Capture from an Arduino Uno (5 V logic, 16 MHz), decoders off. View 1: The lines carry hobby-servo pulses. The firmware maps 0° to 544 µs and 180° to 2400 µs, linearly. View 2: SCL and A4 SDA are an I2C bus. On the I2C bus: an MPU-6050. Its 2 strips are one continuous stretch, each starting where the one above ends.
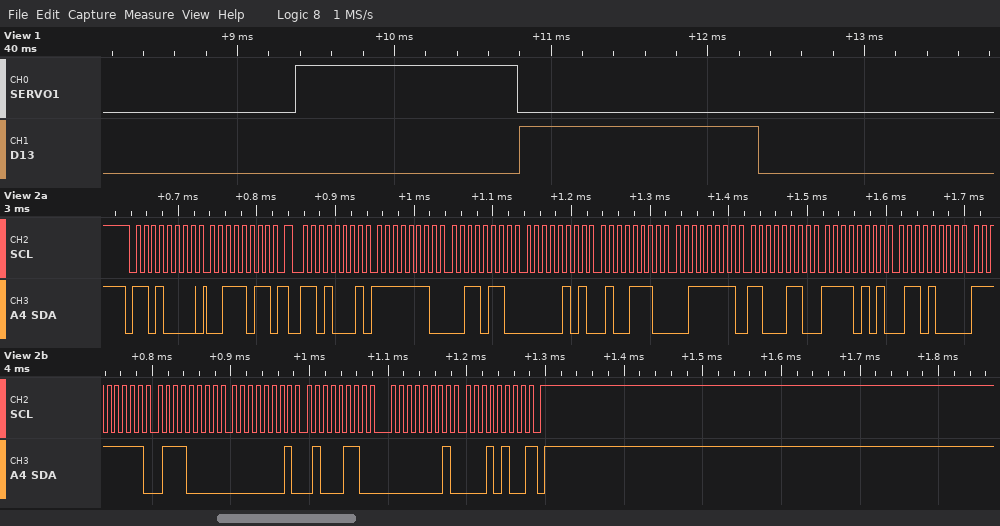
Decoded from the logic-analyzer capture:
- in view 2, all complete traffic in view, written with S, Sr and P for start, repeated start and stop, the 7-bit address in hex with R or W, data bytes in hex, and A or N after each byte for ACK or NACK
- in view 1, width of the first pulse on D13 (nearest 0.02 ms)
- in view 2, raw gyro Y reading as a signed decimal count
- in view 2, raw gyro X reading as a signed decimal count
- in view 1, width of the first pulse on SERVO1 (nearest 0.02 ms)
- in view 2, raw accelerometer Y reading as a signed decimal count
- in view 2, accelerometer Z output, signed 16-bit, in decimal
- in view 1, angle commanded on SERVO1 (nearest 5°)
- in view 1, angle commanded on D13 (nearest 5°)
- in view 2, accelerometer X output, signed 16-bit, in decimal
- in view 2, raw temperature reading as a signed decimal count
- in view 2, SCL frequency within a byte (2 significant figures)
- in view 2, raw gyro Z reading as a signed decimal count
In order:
S 68W A 3B A Sr 68R A FE A 36 A 05 A 4E A 3F A C6 A F5 A 68 A FF A 70 A 01 A 46 A 01 A 14 N P
1.52 ms
326
-144
1.42 ms
1358
16326
85°
95°
-458
-2712
100 kHz
276
